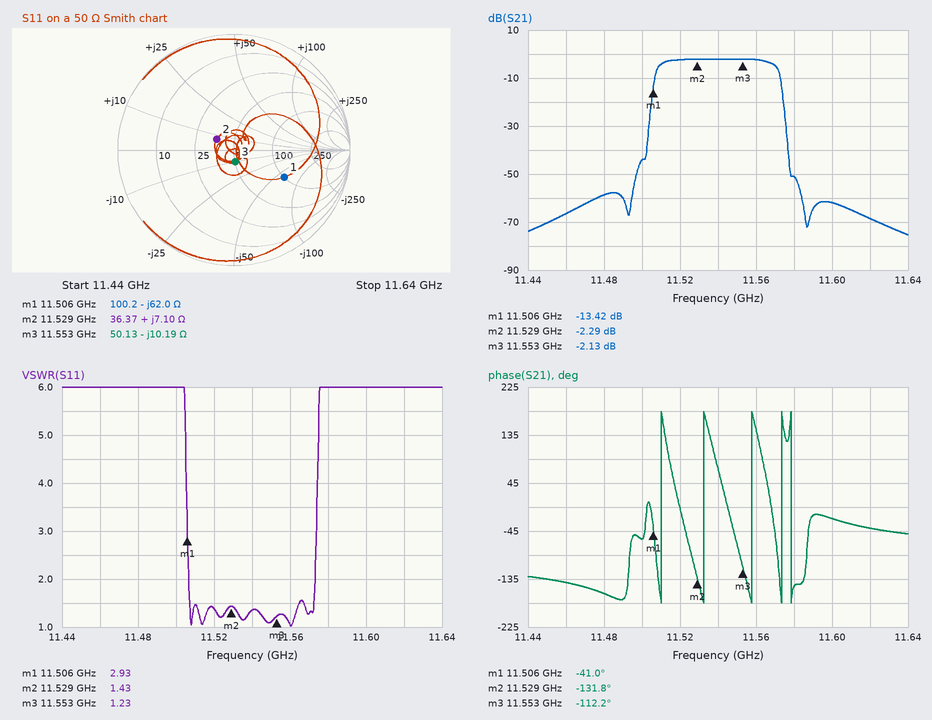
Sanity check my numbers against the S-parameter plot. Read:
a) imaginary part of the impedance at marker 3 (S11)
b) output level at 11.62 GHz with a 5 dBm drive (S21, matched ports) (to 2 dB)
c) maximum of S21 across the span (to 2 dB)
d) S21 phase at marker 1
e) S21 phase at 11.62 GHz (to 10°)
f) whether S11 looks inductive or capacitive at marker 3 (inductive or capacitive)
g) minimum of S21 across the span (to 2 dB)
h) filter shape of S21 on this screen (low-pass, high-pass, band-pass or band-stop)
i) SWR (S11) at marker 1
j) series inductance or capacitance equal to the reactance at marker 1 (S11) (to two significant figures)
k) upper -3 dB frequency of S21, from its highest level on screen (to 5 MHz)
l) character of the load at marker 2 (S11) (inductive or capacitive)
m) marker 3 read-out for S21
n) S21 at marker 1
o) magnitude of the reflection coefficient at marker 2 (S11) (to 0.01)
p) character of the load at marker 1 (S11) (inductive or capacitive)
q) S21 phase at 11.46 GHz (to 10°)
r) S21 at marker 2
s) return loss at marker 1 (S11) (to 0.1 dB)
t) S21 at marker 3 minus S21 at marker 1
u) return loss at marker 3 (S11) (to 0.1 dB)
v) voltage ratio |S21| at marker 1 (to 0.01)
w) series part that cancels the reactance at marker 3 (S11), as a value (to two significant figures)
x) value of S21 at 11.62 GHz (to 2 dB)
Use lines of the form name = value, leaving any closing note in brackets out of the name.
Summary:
imaginary part of the impedance at marker 3 = -10.19 Ω
output level at 11.62 GHz with a 5 dBm drive (S21, matched ports) = -64 dBm
maximum of S21 across the span = -2 dB
S21 phase at marker 1 = -41.0°
S21 phase at 11.62 GHz = -40°
whether S11 looks inductive or capacitive at marker 3 = capacitive
minimum of S21 across the span = -76 dB
filter shape of S21 on this screen = band-pass
SWR (S11) at marker 1 = 2.93
series inductance or capacitance equal to the reactance at marker 1 (S11) = 220 fF
upper -3 dB frequency of S21, from its highest level on screen = 11.570 GHz
character of the load at marker 2 (S11) = inductive
marker 3 read-out for S21 = -2.13 dB
S21 at marker 1 = -13.42 dB
magnitude of the reflection coefficient at marker 2 (S11) = 0.18
character of the load at marker 1 (S11) = capacitive
S21 phase at 11.46 GHz = -140°
S21 at marker 2 = -2.29 dB
return loss at marker 1 (S11) = 6.2 dB
S21 at marker 3 minus S21 at marker 1 = 11.29 dB
return loss at marker 3 (S11) = 19.9 dB
voltage ratio |S21| at marker 1 = 0.21
series part that cancels the reactance at marker 3 (S11), as a value = 140 pH
value of S21 at 11.62 GHz = -68 dB
